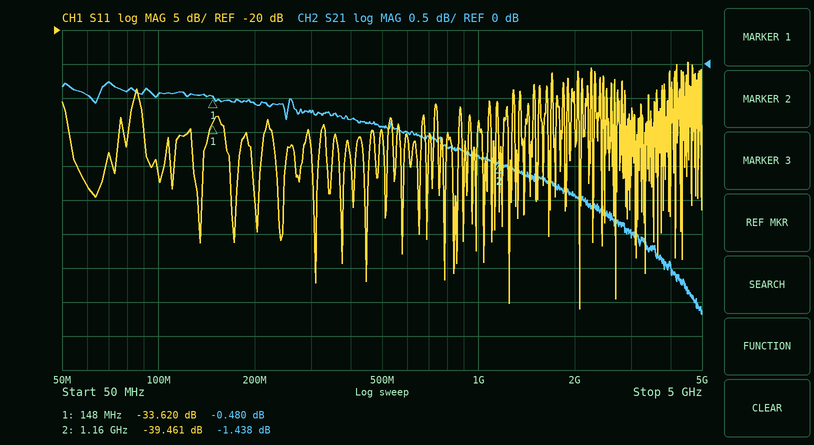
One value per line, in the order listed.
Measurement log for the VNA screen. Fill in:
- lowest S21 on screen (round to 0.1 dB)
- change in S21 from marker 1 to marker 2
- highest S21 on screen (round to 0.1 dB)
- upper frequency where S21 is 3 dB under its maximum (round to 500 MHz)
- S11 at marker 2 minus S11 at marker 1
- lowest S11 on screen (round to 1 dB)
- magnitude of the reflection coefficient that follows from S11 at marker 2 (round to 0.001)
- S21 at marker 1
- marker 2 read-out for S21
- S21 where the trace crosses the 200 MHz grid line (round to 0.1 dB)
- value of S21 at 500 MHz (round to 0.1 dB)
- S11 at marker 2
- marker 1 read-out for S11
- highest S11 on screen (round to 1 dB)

-3.7 dB
-0.958 dB
-0.3 dB
4.5 GHz
-5.841 dB
-61 dB
0.011
-0.480 dB
-1.438 dB
-0.6 dB
-0.9 dB
-39.461 dB
-33.620 dB
-25 dB
